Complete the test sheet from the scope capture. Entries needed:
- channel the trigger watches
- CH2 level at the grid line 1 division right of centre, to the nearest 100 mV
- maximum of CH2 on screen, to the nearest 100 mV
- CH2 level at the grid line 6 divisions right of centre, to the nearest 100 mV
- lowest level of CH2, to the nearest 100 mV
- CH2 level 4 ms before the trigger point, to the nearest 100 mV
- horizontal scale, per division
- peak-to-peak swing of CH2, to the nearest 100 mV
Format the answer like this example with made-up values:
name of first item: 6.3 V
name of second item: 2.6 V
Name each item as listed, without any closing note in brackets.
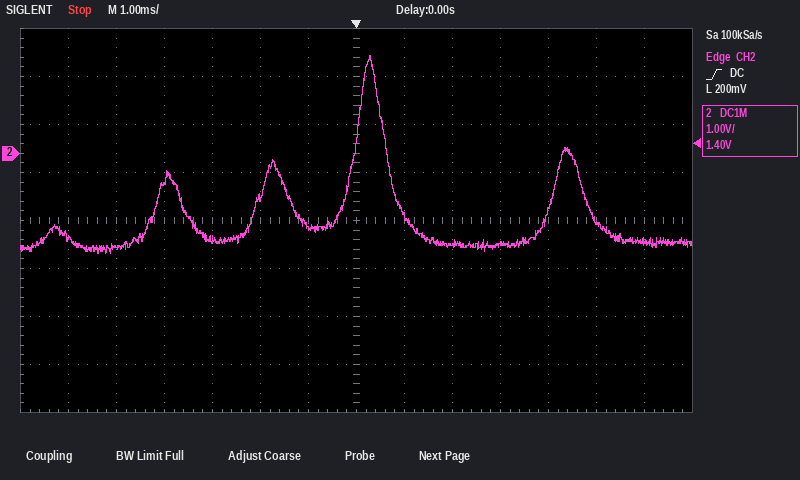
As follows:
channel the trigger watches: CH2
CH2 level at the grid line 1 division right of centre, to the nearest 100 mV: -1.3 V
maximum of CH2 on screen, to the nearest 100 mV: 2.0 V
CH2 level at the grid line 6 divisions right of centre, to the nearest 100 mV: -1.8 V
lowest level of CH2, to the nearest 100 mV: -2.1 V
CH2 level 4 ms before the trigger point, to the nearest 100 mV: -600 mV
horizontal scale, per division: 1 ms
peak-to-peak swing of CH2, to the nearest 100 mV: 4.1 V
